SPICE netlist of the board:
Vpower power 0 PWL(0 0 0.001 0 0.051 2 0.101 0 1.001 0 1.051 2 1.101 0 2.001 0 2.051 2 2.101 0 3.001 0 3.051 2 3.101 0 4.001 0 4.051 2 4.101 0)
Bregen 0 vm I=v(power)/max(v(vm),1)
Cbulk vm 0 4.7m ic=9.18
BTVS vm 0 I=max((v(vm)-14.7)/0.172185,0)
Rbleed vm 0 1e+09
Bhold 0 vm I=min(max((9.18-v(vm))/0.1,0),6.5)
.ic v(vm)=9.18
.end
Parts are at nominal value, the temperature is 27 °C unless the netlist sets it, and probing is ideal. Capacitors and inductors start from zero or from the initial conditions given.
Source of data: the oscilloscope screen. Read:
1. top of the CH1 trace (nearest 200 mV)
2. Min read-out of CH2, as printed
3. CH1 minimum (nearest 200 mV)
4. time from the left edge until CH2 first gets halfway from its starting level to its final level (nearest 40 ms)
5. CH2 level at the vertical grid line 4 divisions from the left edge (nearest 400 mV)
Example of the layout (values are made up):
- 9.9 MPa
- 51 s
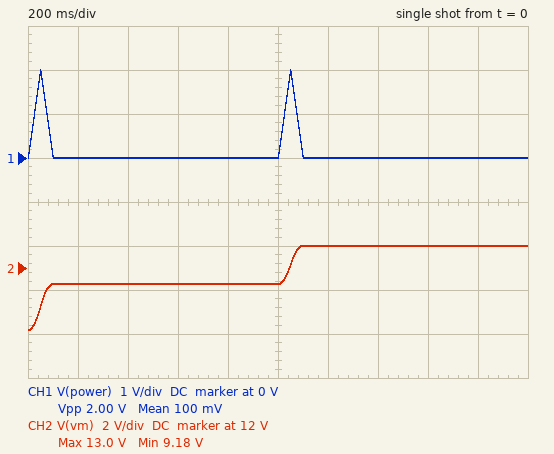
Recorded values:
- 2.0 V
- 9.18 V
- 0 V
- 80 ms
- 11.2 V
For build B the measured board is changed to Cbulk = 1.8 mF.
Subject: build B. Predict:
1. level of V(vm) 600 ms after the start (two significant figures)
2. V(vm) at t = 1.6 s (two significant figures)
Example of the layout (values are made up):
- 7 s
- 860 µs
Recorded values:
- 14 V
- 15 V
